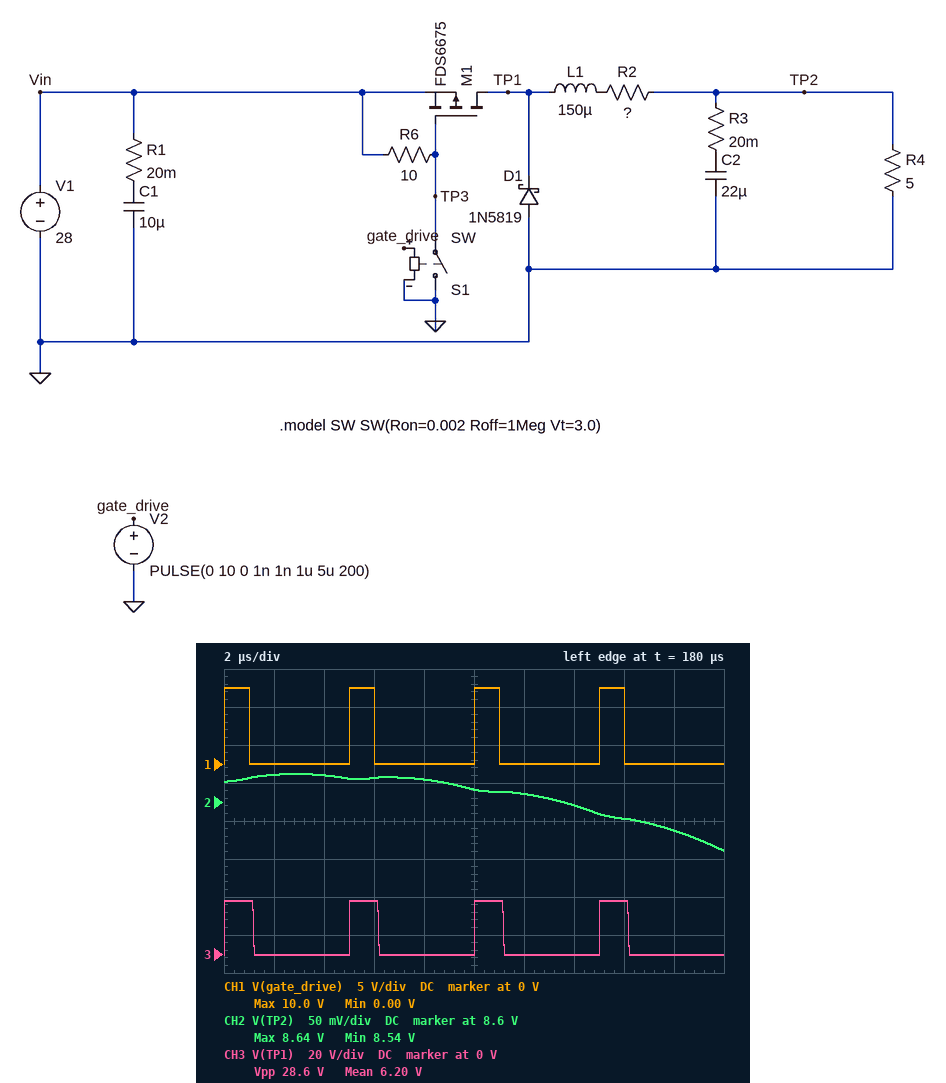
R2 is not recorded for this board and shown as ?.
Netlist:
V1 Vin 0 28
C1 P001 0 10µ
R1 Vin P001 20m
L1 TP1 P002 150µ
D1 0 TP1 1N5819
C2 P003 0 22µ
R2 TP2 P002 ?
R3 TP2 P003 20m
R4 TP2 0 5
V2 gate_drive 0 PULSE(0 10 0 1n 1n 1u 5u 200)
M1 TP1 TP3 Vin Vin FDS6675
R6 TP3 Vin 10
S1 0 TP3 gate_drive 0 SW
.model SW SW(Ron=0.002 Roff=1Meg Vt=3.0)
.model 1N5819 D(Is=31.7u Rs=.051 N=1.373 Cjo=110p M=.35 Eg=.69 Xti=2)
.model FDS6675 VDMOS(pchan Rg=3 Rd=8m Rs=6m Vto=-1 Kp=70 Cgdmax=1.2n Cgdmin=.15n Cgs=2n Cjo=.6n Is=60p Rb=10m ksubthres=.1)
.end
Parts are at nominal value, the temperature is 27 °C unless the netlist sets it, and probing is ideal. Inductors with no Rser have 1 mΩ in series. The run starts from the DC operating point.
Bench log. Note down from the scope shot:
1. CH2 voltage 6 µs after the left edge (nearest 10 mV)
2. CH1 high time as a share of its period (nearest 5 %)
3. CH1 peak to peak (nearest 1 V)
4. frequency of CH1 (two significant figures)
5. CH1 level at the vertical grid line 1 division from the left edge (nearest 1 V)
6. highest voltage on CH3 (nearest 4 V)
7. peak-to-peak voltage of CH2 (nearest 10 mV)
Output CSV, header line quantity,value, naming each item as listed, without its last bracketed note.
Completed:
quantity,value
CH2 voltage 6 µs after the left edge,8.63 V
CH1 high time as a share of its period,20 %
CH1 peak to peak,10 V
frequency of CH1,200 kHz
CH1 level at the vertical grid line 1 division from the left edge,0 V
highest voltage on CH3,28 V
peak-to-peak voltage of CH2,100 mV
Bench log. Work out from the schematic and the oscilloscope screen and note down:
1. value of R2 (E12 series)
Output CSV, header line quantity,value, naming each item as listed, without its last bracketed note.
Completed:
quantity,value
value of R2,0.047 Ω
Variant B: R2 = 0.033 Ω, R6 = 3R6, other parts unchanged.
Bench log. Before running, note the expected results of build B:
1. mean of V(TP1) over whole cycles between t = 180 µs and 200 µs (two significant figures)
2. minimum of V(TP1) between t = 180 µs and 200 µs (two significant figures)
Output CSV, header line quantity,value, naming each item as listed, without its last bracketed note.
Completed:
quantity,value
mean of V(TP1) over whole cycles between t = 180 µs and 200 µs,5.7 V
minimum of V(TP1) between t = 180 µs and 200 µs,-510 mV
